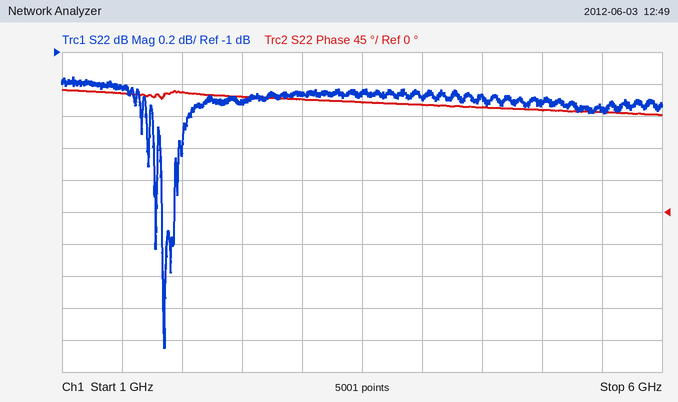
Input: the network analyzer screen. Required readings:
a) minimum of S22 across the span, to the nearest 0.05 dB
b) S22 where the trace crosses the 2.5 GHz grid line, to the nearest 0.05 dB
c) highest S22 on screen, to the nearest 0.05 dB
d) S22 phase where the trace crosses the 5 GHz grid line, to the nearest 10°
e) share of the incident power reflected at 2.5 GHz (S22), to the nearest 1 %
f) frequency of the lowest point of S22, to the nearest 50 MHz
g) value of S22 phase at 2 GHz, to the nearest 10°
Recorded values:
-2.85 dB
-1.30 dB
-1.15 dB
140°
74 %
1.85 GHz
170°
